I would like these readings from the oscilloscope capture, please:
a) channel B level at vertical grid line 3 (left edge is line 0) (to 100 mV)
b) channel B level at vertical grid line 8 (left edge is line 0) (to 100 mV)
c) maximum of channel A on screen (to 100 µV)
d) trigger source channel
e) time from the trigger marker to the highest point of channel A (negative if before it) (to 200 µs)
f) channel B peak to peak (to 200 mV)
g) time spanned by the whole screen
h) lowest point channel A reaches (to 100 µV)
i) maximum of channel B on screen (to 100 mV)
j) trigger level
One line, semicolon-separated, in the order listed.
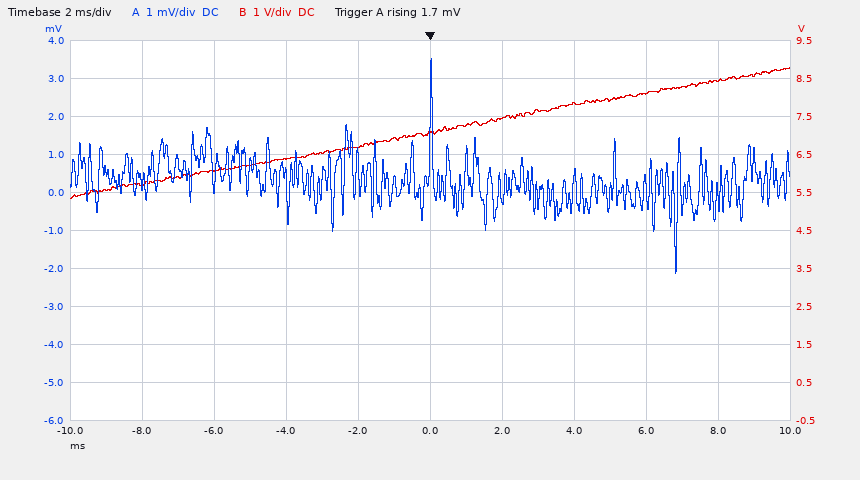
6.4 V; 8.1 V; 3.5 mV; channel A; 0.0 ms; 3.4 V; 20 ms; -2.1 mV; 8.8 V; 1.7 mV
